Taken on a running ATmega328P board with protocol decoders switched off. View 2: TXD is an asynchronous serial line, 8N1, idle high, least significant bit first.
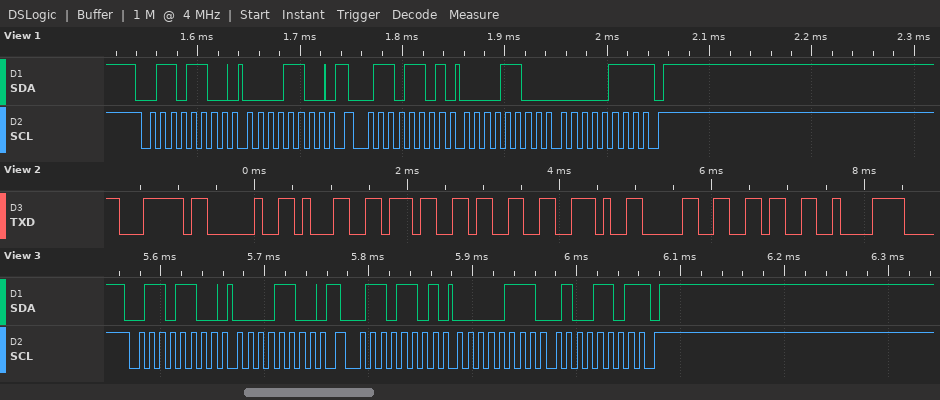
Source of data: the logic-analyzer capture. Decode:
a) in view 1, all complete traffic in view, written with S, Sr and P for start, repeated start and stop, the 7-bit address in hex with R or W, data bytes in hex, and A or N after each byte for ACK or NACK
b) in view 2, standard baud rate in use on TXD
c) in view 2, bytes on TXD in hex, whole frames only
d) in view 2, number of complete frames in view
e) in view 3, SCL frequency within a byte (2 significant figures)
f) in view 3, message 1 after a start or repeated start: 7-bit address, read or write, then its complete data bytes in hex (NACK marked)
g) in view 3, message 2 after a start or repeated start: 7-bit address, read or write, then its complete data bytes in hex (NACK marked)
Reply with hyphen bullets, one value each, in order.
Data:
- S 36W A 0C A Sr 36R A 0C A 07 N P
- 9600 baud
- 7C 20 31 37 33 2E 30 36 C2
- 9
- 100 kHz
- 0x36 write: 0C
- 0x36 read: 07 4D NACK
